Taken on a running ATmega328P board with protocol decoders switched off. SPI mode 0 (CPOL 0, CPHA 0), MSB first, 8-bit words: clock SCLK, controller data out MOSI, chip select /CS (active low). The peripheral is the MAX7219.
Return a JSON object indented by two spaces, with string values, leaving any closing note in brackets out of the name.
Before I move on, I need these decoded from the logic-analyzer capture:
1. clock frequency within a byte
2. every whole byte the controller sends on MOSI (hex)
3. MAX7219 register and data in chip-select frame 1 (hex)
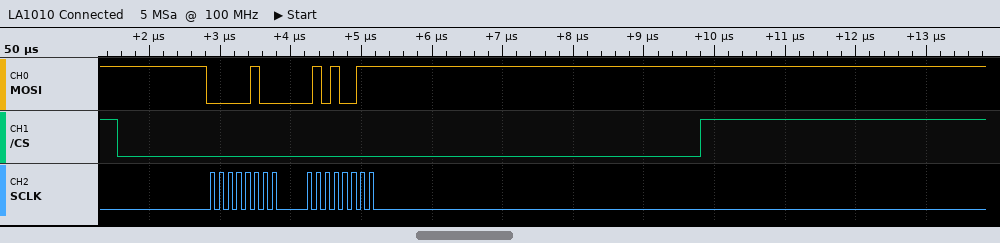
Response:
{
  "clock frequency within a byte": "8 MHz",
  "every whole byte the controller sends on MOSI": "04 53",
  "MAX7219 register and data in chip-select frame 1": "register 0x4, data 0x53"
}
